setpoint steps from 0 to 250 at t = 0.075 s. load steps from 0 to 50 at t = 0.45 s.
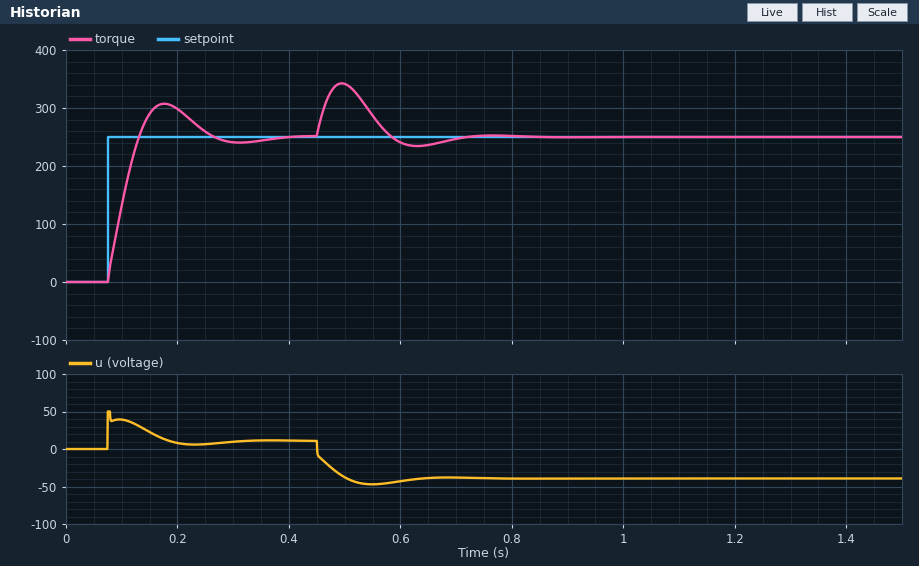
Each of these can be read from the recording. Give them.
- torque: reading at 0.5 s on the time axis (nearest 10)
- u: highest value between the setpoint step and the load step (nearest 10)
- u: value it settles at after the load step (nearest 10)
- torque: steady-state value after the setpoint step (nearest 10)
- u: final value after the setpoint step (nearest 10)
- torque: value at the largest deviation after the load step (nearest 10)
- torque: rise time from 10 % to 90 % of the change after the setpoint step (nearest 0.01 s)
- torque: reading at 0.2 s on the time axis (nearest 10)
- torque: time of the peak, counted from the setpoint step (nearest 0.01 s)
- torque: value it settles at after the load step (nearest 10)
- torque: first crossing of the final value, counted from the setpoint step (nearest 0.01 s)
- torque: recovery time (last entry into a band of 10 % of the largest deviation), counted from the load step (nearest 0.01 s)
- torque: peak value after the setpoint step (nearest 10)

340
50
-40
250
10
340
0.04 s
300
0.10 s
250
0.06 s
0.22 s
310
